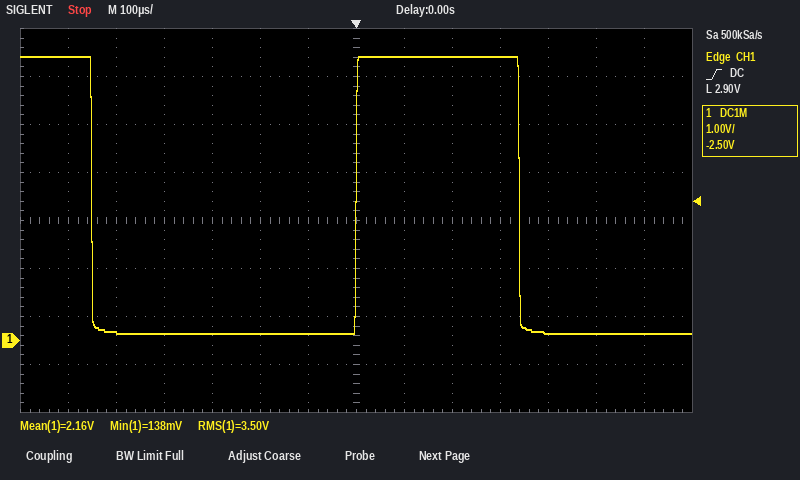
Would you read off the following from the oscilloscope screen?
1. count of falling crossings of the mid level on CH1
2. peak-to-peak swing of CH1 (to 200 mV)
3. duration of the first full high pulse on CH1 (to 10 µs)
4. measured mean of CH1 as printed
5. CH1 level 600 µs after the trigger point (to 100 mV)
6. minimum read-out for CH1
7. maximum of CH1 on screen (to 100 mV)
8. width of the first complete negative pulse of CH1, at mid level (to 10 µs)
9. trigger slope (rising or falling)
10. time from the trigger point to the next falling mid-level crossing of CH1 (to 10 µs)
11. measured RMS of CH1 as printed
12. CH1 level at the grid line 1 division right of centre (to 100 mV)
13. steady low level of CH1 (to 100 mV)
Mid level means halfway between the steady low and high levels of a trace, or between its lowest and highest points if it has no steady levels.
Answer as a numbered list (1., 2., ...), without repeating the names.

1. 2
2. 5.8 V
3. 340 µs
4. 2.16 V
5. 100 mV
6. 138 mV
7. 5.9 V
8. 550 µs
9. rising
10. 340 µs
11. 3.50 V
12. 5.9 V
13. 100 mV
